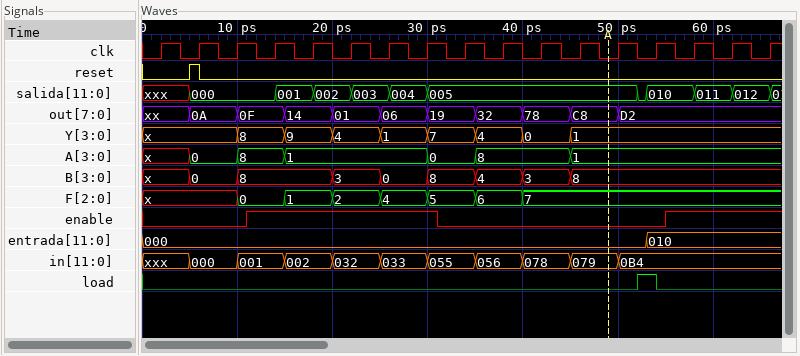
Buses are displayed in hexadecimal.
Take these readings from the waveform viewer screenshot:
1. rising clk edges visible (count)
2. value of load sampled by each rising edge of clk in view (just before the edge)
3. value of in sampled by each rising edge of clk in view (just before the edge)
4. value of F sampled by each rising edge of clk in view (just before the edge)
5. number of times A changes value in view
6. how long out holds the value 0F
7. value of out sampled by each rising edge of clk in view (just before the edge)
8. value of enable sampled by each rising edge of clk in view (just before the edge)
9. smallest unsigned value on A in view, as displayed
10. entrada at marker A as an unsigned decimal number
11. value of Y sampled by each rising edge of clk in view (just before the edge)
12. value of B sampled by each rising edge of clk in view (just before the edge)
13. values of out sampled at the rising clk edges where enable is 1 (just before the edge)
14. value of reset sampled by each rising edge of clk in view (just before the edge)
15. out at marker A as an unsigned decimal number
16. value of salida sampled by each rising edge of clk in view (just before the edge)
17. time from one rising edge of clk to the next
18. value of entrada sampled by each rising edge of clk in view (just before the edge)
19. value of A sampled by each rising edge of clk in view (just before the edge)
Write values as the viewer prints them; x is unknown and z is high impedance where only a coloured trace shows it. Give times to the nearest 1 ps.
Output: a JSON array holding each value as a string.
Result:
["17", "0 0 0 0 0 0 0 0 0 0 0 0 0 1 0 0 0", "xxx, 000, 000, 001, 002, 032, 033, 033, 055, 056, 078, 079, 079, 0B4, 0B4, 0B4, 0B4", "x, x, x, 0, 1, 2, 4, 4, 5, 6, 7, 7, 7, 7, 7, 7, 7", "6", "5 ps", "xx, 0A, 0A, 0F, 14, 01, 06, 06, 19, 32, 78, C8, C8, D2, D2, D2, D2", "0 0 0 1 1 1 1 1 0 0 0 0 0 0 1 1 1", "0", "0", "x, x, x, 8, 9, 4, 1, 1, 7, 4, 0, 1, 1, 1, 1, 1, 1", "x, 0, 0, 8, 8, 3, 0, 0, 8, 4, 3, 8, 8, 8, 8, 8, 8", "0F, 14, 01, 06, 06, D2, D2, D2", "0 1 0 0 0 0 0 0 0 0 0 0 0 0 0 0 0", "200", "xxx, 000, 000, 000, 001, 002, 003, 004, 005, 005, 005, 005, 005, 010, 010, 011, 012", "4 ps", "000, 000, 000, 000, 000, 000, 000, 000, 000, 000, 000, 000, 000, 010, 010, 010, 010", "x, 0, 0, 8, 1, 1, 1, 1, 0, 8, 8, 1, 1, 1, 1, 1, 1"]
